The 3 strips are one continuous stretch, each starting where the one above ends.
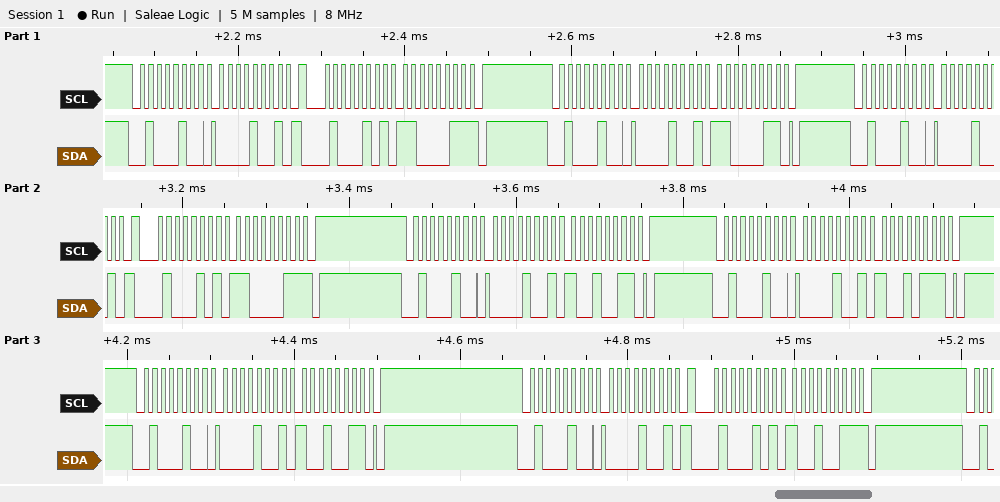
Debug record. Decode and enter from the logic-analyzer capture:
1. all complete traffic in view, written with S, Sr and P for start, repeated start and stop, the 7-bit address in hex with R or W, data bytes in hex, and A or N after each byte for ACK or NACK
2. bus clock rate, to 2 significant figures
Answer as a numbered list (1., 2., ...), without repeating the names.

1. S 22W A 09 A Sr 22R A C3 N P S 22W A 09 A C3 A P S 22W A 09 A Sr 22R A C3 N P S 22W A 09 A 93 A P S 22W A 09 A 97 A P S 22W A 09 A 93 A P S 22W A 09 A Sr 22R A 93 N P
2. 100 kHz
